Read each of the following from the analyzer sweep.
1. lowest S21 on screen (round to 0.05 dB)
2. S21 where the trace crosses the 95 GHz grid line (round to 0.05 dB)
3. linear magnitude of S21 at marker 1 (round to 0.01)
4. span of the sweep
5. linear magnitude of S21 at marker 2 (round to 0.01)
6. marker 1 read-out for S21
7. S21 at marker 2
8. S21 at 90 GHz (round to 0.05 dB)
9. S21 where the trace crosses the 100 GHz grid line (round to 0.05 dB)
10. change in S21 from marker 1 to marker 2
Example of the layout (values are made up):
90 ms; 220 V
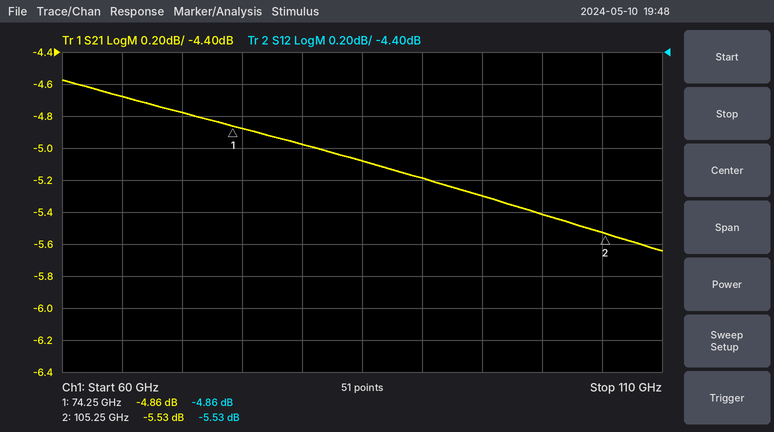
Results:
-5.65 dB; -5.30 dB; 0.57; 50 GHz; 0.53; -4.86 dB; -5.53 dB; -5.20 dB; -5.40 dB; -0.67 dB
